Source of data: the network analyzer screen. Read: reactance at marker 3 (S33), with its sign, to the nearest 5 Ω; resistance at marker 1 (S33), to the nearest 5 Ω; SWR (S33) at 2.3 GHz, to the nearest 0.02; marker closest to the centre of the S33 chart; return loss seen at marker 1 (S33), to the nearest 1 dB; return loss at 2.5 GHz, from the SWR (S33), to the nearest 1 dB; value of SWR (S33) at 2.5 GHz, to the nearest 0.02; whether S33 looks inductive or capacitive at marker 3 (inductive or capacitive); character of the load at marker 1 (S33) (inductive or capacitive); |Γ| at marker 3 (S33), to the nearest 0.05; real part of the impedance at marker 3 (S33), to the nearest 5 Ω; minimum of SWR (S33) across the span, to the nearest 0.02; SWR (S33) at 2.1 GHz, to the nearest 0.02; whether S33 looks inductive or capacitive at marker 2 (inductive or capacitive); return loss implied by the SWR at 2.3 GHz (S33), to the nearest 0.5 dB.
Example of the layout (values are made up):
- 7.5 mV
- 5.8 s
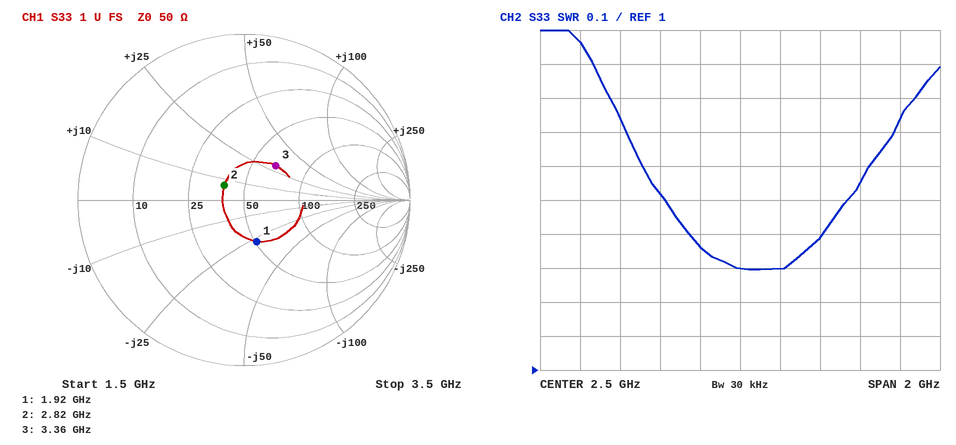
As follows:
- +30 Ω
- 50 Ω
- 1.36
- marker 2
- 12 dB
- 18 dB
- 1.30
- inductive
- capacitive
- 0.30
- 65 Ω
- 1.30
- 1.52
- inductive
- 16.5 dB
